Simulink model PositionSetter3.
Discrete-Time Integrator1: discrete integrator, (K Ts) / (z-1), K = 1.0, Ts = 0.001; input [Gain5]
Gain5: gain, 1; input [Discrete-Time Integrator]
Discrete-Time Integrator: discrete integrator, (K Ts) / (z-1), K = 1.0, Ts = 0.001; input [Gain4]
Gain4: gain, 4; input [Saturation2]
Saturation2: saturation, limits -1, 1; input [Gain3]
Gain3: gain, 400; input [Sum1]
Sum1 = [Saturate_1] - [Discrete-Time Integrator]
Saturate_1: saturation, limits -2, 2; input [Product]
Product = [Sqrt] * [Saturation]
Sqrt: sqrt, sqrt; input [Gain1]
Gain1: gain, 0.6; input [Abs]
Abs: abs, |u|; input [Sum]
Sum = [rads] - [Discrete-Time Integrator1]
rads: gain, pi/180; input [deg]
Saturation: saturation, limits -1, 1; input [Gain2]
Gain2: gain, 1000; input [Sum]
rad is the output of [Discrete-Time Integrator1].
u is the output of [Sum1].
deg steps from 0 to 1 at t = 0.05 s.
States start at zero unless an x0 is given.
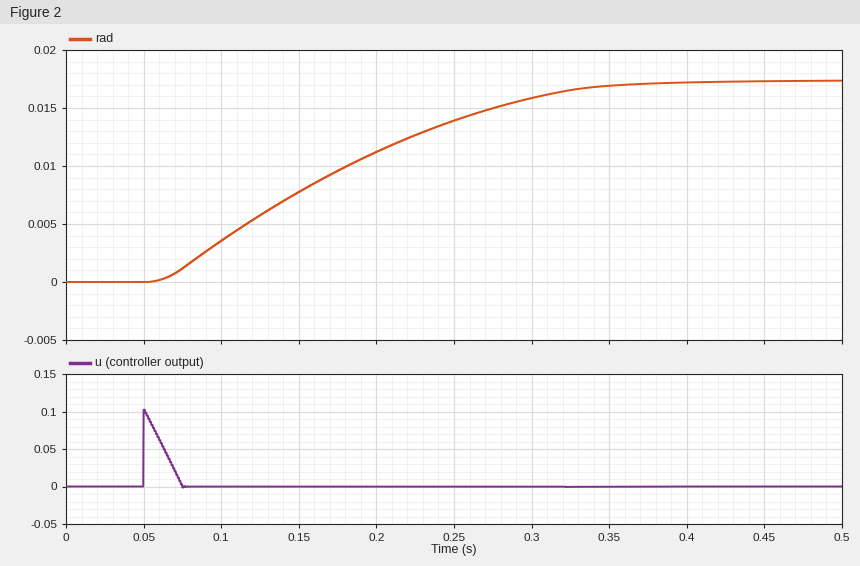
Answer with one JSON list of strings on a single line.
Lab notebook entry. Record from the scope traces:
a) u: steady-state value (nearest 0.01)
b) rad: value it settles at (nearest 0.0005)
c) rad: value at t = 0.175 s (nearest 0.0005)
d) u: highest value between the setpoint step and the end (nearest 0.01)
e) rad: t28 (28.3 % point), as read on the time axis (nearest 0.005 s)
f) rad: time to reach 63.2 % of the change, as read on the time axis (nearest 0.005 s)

["0.00", "0.0175", "0.0095", "0.10", "0.115 s", "0.195 s"]
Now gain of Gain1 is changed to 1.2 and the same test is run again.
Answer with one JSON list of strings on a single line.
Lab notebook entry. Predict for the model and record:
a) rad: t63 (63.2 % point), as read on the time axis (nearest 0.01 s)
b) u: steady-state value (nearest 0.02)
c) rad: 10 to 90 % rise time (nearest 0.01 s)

["0.16 s", "0.00", "0.15 s"]
